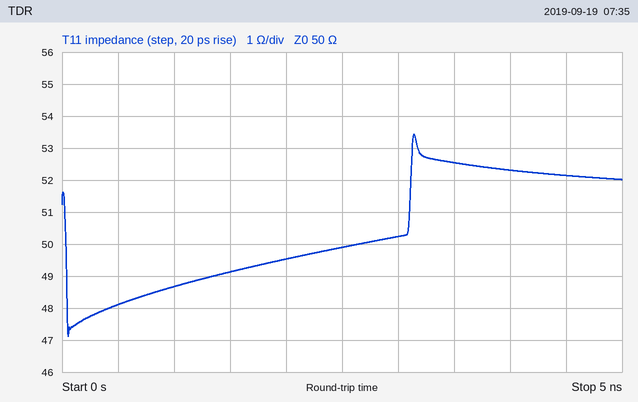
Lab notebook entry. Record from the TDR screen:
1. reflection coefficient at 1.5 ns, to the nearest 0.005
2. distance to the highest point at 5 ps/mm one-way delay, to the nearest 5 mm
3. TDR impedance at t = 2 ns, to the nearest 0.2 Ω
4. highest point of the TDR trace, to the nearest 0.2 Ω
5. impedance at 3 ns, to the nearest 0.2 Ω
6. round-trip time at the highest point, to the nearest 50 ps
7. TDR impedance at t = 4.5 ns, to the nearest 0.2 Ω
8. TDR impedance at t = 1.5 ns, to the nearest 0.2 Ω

-0.010
315 mm
49.6 Ω
53.4 Ω
50.2 Ω
3.15 ns
52.2 Ω
49.2 Ω
